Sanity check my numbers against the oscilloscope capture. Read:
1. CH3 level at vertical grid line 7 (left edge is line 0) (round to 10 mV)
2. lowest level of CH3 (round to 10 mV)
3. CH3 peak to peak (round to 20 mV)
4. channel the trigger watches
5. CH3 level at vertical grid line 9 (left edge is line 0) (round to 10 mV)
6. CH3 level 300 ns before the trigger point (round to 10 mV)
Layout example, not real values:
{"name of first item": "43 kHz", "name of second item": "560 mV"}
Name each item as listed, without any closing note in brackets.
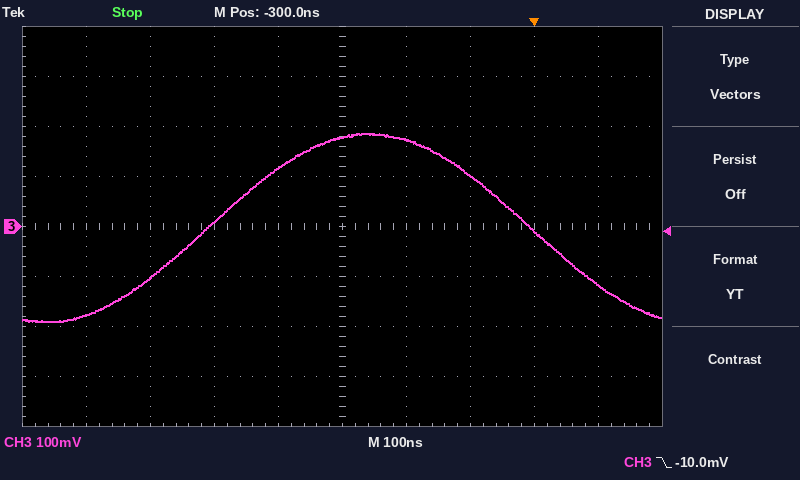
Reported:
{"CH3 level at vertical grid line 7 (left edge is line 0)": "100 mV", "lowest level of CH3": "-190 mV", "CH3 peak to peak": "380 mV", "channel the trigger watches": "CH3", "CH3 level at vertical grid line 9 (left edge is line 0)": "-120 mV", "CH3 level 300 ns before the trigger point": "180 mV"}
